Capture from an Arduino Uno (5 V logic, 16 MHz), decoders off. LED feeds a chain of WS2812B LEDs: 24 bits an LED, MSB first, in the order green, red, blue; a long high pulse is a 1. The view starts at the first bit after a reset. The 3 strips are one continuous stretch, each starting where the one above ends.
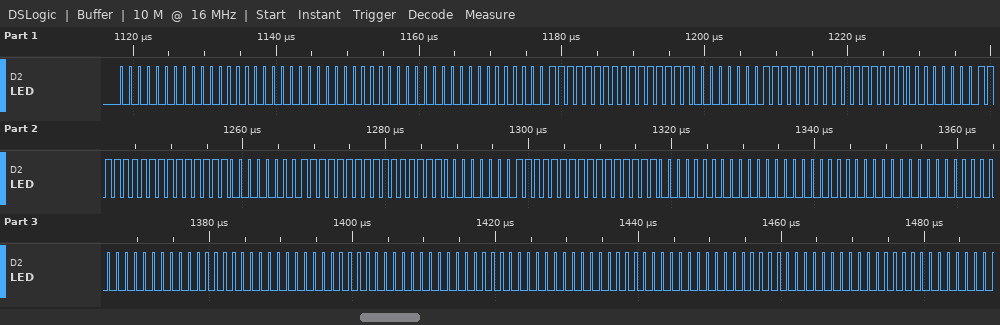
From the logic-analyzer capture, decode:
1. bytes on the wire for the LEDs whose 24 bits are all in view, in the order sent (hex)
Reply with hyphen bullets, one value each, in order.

- 00 00 00 00 00 00 FF FF 00 FF FF 00 FF FF 00 FF FF 00 FF FF 00 00 00 00 00 00 00 00 00 00 00 00 00 00 00 00
